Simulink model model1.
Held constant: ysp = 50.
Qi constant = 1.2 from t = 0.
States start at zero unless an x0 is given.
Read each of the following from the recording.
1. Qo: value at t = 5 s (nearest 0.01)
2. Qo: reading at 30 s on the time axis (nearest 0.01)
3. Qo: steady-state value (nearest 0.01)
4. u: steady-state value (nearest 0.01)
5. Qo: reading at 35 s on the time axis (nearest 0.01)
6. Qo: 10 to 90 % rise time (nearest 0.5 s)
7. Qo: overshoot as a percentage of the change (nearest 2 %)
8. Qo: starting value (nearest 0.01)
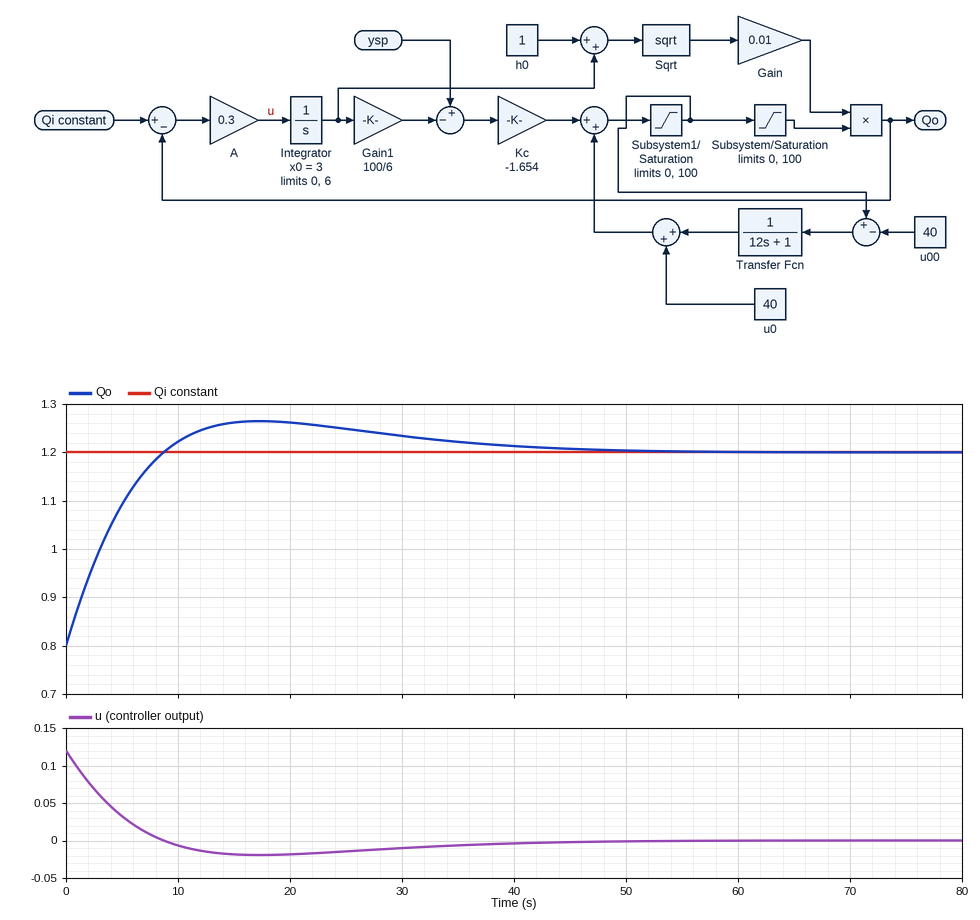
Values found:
1.09
1.23
1.20
0.00
1.22
6.5 s
16 %
0.80
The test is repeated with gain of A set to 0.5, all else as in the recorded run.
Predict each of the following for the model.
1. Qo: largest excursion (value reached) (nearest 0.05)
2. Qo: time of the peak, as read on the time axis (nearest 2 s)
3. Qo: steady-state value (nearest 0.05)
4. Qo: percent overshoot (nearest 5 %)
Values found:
1.25
12 s
1.20
10 %
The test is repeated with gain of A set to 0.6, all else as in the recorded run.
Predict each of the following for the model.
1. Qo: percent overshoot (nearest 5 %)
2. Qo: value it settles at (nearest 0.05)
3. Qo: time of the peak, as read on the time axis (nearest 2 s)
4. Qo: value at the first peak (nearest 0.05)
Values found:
10 %
1.20
10 s
1.25
